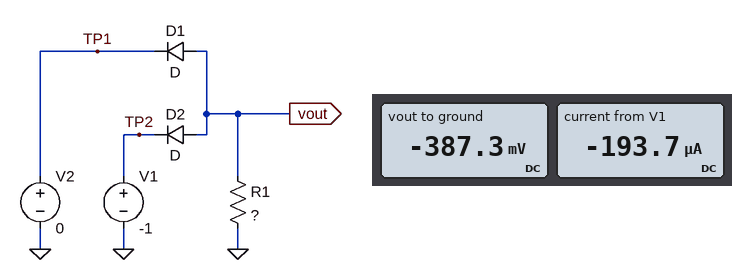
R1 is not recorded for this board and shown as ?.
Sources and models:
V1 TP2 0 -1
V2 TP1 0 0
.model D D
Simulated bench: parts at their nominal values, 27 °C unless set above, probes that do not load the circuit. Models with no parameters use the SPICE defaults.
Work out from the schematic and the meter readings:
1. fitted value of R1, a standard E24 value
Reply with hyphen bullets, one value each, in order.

- 2 kΩ
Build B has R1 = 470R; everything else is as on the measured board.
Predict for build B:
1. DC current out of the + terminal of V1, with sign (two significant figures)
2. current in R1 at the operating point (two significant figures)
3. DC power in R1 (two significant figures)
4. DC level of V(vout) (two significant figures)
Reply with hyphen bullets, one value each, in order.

- -750 µA
- 750 µA
- 260 µW
- -350 mV
